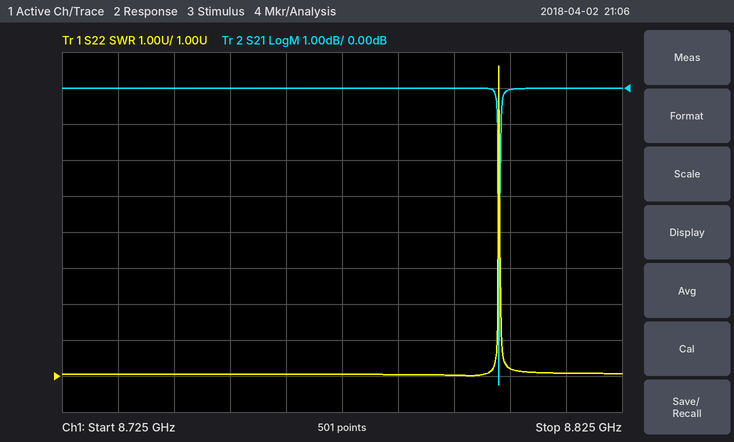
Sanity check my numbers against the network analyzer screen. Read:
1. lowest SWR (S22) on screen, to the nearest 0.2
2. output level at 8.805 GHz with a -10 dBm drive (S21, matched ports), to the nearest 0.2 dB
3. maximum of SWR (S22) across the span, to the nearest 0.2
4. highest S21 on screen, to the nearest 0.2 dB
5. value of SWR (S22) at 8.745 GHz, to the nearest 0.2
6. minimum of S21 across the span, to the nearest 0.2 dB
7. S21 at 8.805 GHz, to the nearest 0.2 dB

1.0
-10.0 dBm
9.6
0.0 dB
1.0
-8.2 dB
0.0 dB
